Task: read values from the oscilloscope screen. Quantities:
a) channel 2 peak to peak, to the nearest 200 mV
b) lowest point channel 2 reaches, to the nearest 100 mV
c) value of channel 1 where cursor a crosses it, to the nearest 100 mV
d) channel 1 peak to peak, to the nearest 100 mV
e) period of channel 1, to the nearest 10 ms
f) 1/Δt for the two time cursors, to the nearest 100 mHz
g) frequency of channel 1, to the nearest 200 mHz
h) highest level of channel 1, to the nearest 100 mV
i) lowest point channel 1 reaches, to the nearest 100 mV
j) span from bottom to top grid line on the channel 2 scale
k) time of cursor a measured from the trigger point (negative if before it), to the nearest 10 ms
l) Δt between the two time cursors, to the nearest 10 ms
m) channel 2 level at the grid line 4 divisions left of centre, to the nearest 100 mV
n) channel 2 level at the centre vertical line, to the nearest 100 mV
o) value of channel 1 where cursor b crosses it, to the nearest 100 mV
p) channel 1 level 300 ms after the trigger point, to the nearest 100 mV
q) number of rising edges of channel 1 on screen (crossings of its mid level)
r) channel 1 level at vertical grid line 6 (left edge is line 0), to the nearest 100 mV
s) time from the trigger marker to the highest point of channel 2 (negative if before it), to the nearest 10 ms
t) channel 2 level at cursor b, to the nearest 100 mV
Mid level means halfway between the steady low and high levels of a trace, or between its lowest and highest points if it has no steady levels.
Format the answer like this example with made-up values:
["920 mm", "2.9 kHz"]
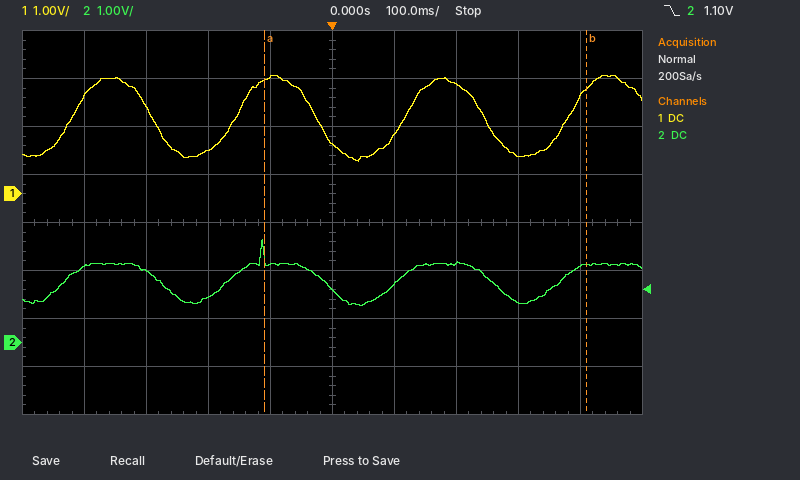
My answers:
["1.4 V", "800 mV", "2.4 V", "1.8 V", "270 ms", "1.9 Hz", "3.8 Hz", "2.5 V", "700 mV", "8 V", "-110 ms", "520 ms", "1.6 V", "1.1 V", "2.2 V", "800 mV", "4", "1.2 V", "-110 ms", "1.6 V"]
